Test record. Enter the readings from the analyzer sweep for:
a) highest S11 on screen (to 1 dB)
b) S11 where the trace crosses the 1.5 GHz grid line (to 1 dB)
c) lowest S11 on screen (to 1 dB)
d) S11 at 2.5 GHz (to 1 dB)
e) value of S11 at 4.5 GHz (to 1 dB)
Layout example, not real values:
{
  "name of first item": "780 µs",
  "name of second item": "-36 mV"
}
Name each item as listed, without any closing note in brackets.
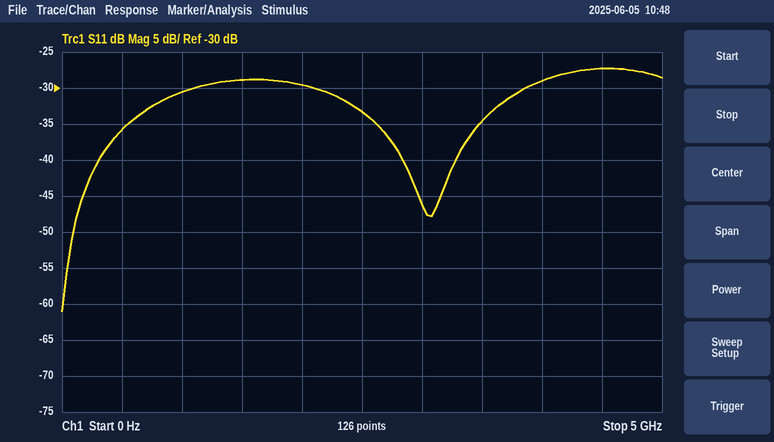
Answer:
{
  "highest S11 on screen": "-27 dB",
  "S11 where the trace crosses the 1.5 GHz grid line": "-29 dB",
  "lowest S11 on screen": "-61 dB",
  "S11 at 2.5 GHz": "-33 dB",
  "value of S11 at 4.5 GHz": "-27 dB"
}
